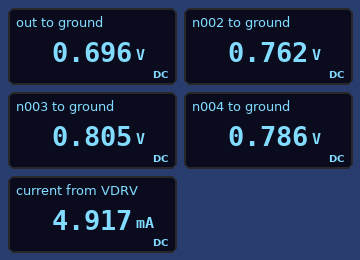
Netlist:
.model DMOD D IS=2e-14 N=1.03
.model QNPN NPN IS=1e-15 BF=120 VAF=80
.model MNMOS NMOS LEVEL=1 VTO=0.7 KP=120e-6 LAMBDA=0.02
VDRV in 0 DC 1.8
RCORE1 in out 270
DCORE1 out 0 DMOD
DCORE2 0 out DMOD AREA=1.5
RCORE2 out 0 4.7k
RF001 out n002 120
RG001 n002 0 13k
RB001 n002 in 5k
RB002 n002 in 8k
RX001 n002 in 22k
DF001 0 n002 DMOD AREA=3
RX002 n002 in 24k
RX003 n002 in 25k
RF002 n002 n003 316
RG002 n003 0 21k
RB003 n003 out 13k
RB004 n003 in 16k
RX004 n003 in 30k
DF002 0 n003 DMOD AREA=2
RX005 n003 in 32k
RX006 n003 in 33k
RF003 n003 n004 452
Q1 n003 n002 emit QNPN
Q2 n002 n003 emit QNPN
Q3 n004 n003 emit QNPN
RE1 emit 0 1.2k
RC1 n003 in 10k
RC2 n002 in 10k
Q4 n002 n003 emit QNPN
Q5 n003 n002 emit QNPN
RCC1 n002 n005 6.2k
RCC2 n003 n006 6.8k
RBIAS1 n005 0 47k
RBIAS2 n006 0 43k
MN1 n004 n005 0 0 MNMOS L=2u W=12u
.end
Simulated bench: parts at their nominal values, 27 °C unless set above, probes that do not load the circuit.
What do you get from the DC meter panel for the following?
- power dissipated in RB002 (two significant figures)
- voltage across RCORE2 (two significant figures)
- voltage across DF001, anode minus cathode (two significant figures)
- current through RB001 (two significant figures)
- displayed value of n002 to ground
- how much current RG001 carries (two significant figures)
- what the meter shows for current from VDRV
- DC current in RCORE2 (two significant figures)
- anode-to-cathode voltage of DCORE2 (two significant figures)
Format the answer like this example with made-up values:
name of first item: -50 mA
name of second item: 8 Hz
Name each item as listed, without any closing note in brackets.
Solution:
power dissipated in RB002: 130 µW
voltage across RCORE2: 700 mV
voltage across DF001, anode minus cathode: -760 mV
current through RB001: 210 µA
displayed value of n002 to ground: 0.762 V
how much current RG001 carries: 59 µA
what the meter shows for current from VDRV: 4.917 mA
DC current in RCORE2: 150 µA
anode-to-cathode voltage of DCORE2: -700 mV
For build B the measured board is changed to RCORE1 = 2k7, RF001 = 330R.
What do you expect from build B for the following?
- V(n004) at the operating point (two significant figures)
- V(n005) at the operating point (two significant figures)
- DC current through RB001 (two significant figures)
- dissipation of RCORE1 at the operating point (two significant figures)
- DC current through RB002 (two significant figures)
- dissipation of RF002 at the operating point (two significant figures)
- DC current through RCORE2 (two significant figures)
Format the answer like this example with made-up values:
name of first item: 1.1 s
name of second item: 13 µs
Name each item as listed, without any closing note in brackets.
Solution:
V(n004) at the operating point: 820 mV
V(n005) at the operating point: 710 mV
DC current through RB001: 200 µA
dissipation of RCORE1 at the operating point: 490 µW
DC current through RB002: 120 µA
dissipation of RF002 at the operating point: 3.2 µW
DC current through RCORE2: 140 µA
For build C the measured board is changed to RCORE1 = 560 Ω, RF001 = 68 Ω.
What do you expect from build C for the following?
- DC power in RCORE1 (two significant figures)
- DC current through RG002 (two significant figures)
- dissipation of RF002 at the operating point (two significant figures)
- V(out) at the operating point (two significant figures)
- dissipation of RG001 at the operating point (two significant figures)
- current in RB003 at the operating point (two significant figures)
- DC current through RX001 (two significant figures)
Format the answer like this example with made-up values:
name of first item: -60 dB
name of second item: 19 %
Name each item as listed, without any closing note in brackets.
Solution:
DC power in RCORE1: 2.2 mW
DC current through RG002: 37 µA
dissipation of RF002 at the operating point: 7.9 µW
V(out) at the operating point: 680 mV
dissipation of RG001 at the operating point: 40 µW
current in RB003 at the operating point: 7.0 µA
DC current through RX001: 49 µA
